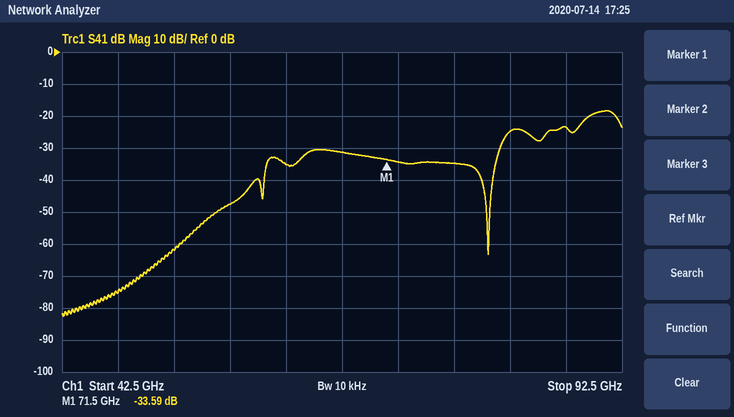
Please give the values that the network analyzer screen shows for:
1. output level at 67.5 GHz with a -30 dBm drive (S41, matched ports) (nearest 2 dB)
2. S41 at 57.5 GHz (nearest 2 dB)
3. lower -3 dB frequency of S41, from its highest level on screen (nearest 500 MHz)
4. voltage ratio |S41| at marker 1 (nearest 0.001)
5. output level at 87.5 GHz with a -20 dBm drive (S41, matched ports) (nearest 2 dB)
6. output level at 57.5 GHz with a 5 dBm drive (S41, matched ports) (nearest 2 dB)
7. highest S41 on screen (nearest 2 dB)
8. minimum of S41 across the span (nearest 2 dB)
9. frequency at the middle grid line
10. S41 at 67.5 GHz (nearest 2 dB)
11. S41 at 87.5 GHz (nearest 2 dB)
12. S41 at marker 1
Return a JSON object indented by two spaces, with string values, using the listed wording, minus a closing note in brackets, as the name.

{
  "output level at 67.5 GHz with a -30 dBm drive (S41, matched ports)": "-62 dBm",
  "S41 at 57.5 GHz": "-48 dB",
  "lower -3 dB frequency of S41, from its highest level on screen": "89.0 GHz",
  "voltage ratio |S41| at marker 1": "0.021",
  "output level at 87.5 GHz with a -20 dBm drive (S41, matched ports)": "-44 dBm",
  "output level at 57.5 GHz with a 5 dBm drive (S41, matched ports)": "-42 dBm",
  "highest S41 on screen": "-18 dB",
  "minimum of S41 across the span": "-82 dB",
  "frequency at the middle grid line": "67.5 GHz",
  "S41 at 67.5 GHz": "-32 dB",
  "S41 at 87.5 GHz": "-24 dB",
  "S41 at marker 1": "-33.59 dB"
}
